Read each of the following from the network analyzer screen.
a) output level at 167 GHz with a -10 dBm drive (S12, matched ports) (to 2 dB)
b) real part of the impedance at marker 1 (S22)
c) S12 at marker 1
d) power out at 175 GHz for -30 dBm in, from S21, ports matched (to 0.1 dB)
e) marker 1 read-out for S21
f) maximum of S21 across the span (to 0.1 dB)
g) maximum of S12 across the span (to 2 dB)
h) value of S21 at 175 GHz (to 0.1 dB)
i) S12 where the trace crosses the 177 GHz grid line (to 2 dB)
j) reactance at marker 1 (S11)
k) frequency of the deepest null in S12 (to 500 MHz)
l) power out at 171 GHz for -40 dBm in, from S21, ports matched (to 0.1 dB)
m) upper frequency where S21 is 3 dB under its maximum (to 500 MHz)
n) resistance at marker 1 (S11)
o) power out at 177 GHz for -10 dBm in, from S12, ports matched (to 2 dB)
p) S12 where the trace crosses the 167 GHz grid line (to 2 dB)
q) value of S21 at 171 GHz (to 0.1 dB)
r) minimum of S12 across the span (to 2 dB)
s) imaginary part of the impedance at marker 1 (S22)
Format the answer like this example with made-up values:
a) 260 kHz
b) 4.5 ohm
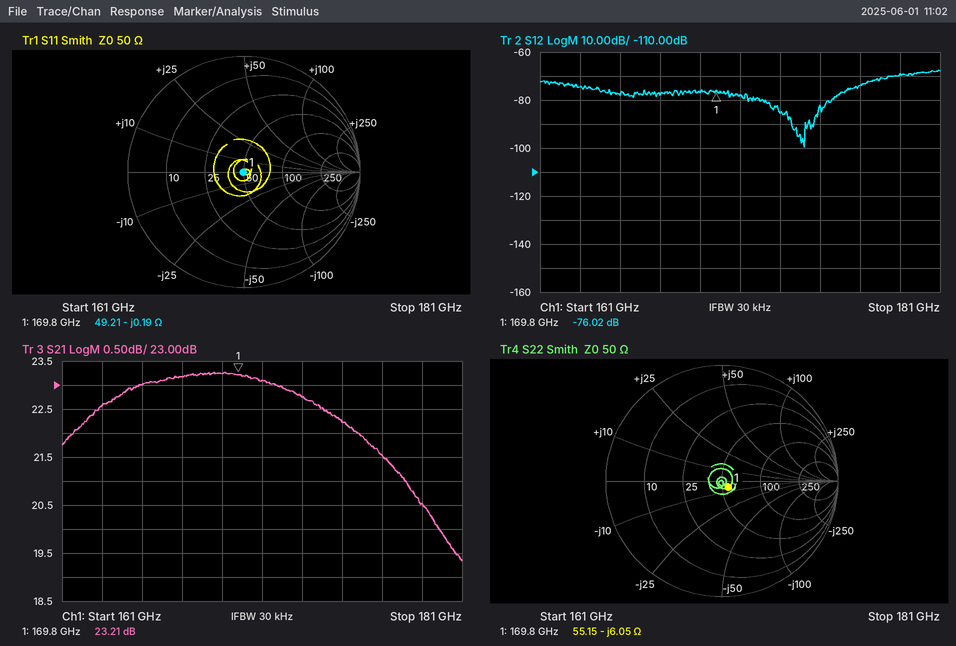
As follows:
a) -88 dBm
b) 55.15 Ω
c) -76.02 dB
d) -7.8 dBm
e) 23.21 dB
f) 23.3 dB
g) -68 dB
h) 22.2 dB
i) -74 dB
j) -0.19 Ω
k) 174.0 GHz
l) -16.9 dBm
m) 179.5 GHz
n) 49.21 Ω
o) -84 dBm
p) -78 dB
q) 23.1 dB
r) -100 dB
s) -6.05 Ω
